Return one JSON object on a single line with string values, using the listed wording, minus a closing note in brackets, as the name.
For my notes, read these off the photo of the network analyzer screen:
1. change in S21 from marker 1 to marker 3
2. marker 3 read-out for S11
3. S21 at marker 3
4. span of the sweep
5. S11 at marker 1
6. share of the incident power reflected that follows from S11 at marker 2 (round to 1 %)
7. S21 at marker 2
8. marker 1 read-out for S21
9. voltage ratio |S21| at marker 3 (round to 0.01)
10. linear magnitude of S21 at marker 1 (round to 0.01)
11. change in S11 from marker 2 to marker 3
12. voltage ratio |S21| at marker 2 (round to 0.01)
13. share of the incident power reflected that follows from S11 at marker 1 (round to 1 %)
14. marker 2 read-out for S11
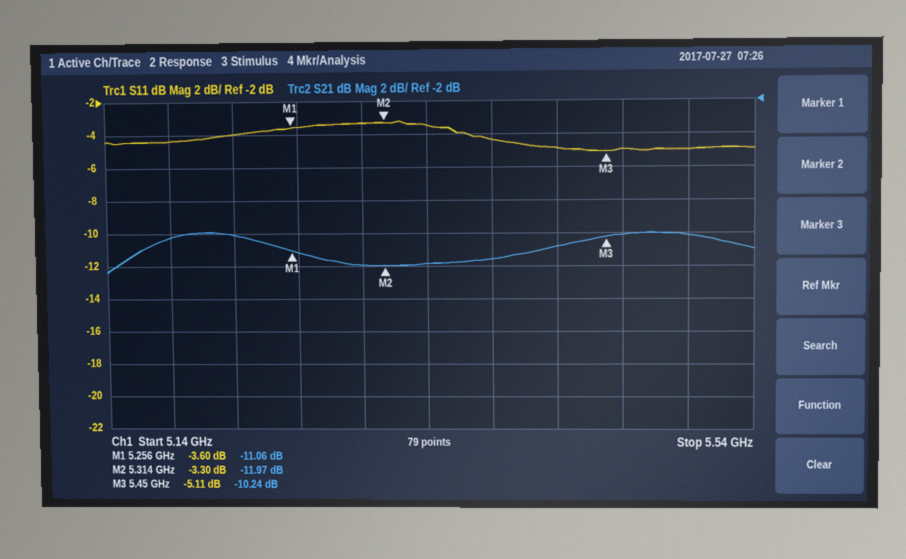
{"change in S21 from marker 1 to marker 3": "0.82 dB", "marker 3 read-out for S11": "-5.11 dB", "S21 at marker 3": "-10.24 dB", "span of the sweep": "400 MHz", "S11 at marker 1": "-3.60 dB", "share of the incident power reflected that follows from S11 at marker 2": "47 %", "S21 at marker 2": "-11.97 dB", "marker 1 read-out for S21": "-11.06 dB", "voltage ratio |S21| at marker 3": "0.31", "linear magnitude of S21 at marker 1": "0.28", "change in S11 from marker 2 to marker 3": "-1.81 dB", "voltage ratio |S21| at marker 2": "0.25", "share of the incident power reflected that follows from S11 at marker 1": "44 %", "marker 2 read-out for S11": "-3.30 dB"}
